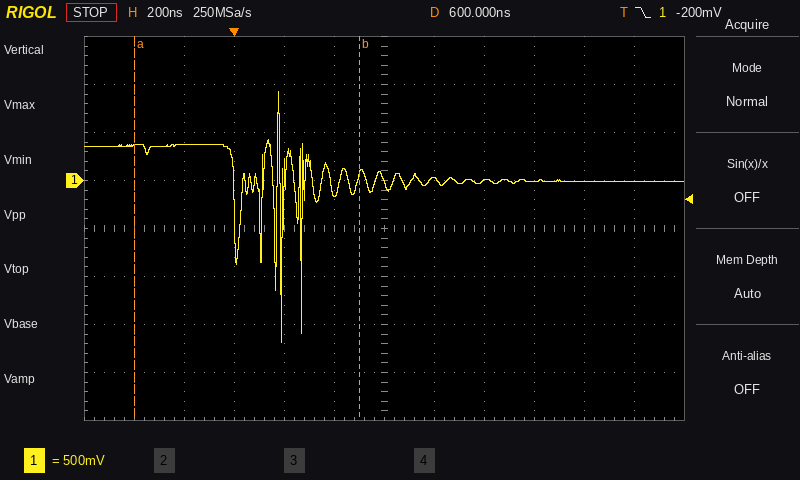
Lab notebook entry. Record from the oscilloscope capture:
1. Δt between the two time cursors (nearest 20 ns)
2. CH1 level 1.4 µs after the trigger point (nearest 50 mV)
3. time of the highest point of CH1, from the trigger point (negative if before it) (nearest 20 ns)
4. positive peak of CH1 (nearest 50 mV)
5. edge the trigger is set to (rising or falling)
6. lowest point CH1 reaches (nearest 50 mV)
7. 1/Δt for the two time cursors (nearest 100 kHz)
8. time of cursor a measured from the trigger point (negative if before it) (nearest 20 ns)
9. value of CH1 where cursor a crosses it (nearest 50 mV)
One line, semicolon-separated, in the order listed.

900 ns; 0 mV; +180 ns; 950 mV; falling; -1.70 V; 1.1 MHz; -400 ns; 350 mV
